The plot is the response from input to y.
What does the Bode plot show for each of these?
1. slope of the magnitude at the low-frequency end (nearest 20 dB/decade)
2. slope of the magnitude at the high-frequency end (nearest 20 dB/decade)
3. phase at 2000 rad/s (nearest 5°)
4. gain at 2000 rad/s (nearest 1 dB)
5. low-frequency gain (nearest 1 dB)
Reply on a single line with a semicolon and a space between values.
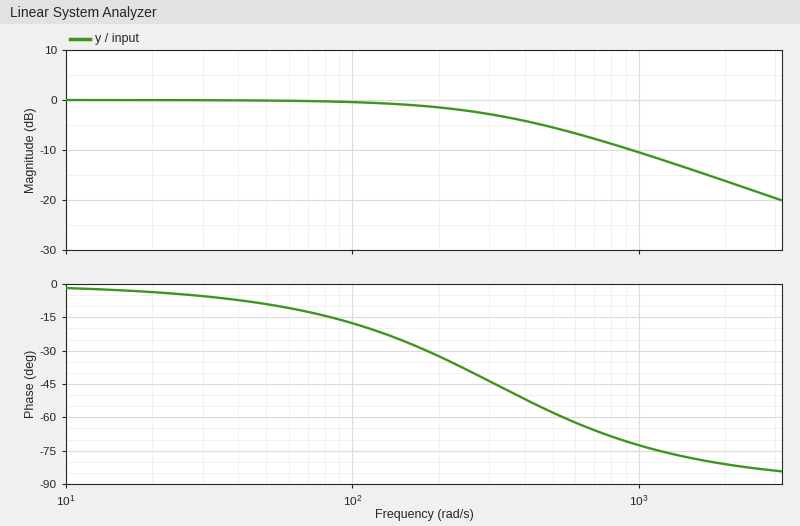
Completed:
0 dB/decade; -20 dB/decade; -80°; -16 dB; 0 dB
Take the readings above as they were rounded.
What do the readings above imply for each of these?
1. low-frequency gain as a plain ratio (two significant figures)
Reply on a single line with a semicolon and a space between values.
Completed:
1.0
